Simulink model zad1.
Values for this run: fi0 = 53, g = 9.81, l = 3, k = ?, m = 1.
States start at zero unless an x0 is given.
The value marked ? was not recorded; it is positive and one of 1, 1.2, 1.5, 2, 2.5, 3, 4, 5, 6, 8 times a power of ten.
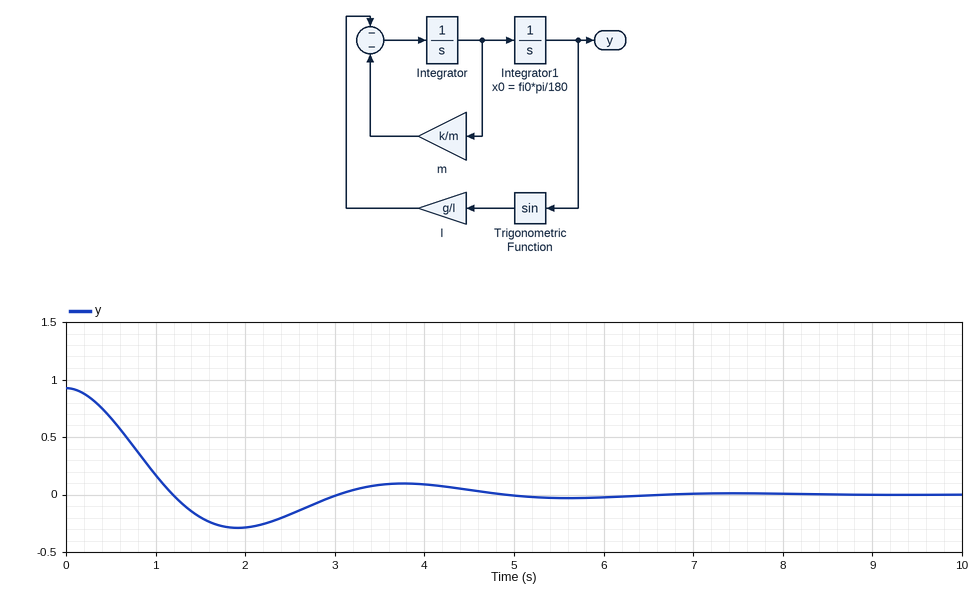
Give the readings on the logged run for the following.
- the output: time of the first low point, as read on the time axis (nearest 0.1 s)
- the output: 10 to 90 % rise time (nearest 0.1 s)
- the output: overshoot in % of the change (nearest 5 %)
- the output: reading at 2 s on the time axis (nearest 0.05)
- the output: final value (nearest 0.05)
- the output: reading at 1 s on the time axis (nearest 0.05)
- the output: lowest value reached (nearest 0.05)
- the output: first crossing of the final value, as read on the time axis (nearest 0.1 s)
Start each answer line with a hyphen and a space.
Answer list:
- 1.9 s
- 0.8 s
- 30 %
- -0.30
- 0.00
- 0.15
- -0.30
- 1.2 s
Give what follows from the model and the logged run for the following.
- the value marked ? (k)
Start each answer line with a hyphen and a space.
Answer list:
- 1.2
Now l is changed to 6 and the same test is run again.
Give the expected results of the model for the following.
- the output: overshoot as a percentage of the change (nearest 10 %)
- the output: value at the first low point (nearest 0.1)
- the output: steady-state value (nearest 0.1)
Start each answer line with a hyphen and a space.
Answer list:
- 20 %
- -0.2
- 0.0
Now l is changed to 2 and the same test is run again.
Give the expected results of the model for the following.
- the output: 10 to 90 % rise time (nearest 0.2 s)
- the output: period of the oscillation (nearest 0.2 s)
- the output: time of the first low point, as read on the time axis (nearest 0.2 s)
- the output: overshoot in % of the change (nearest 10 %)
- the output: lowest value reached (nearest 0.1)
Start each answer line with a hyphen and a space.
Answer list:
- 0.6 s
- 3.0 s
- 1.6 s
- 40 %
- -0.4
